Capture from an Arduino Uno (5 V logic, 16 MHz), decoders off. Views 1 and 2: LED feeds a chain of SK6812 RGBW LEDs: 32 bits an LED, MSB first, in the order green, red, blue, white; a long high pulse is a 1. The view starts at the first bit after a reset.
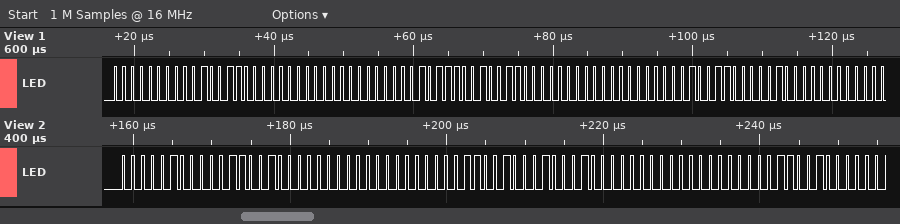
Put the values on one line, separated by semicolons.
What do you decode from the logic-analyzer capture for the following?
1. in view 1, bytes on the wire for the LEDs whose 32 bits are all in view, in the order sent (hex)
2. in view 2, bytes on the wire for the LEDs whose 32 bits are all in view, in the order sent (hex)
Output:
00 26 00 00 17 26 00 00; 04 19 00 00 19 11 00 00
